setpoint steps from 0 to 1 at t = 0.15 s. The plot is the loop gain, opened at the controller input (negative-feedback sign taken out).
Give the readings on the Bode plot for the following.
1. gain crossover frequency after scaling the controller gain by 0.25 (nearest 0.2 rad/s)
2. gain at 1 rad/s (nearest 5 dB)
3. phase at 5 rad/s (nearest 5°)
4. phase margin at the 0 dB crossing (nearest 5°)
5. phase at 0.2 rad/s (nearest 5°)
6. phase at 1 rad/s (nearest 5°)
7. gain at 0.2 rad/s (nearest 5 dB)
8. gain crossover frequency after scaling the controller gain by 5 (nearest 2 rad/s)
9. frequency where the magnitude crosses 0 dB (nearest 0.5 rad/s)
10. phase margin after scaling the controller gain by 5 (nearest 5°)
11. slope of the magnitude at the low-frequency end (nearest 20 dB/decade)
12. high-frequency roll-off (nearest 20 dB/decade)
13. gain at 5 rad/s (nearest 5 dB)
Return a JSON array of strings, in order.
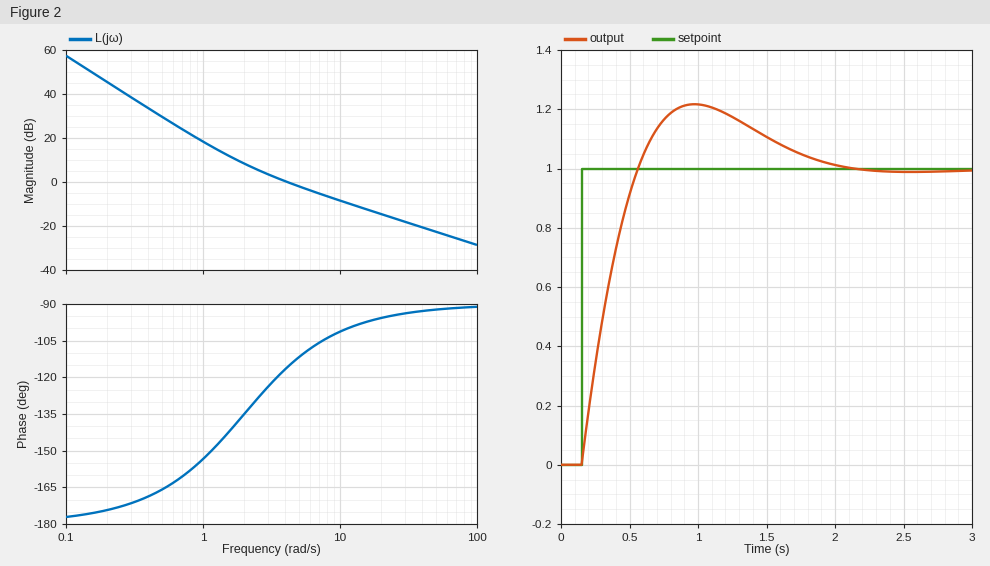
["1.6 rad/s", "20 dB", "-110°", "65°", "-175°", "-155°", "45 dB", "18 rad/s", "4.0 rad/s", "85°", "-40 dB/decade", "-20 dB/decade", "0 dB"]
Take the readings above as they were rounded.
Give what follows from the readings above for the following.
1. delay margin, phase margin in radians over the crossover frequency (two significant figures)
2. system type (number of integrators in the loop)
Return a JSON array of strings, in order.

["0.28 s", "2"]
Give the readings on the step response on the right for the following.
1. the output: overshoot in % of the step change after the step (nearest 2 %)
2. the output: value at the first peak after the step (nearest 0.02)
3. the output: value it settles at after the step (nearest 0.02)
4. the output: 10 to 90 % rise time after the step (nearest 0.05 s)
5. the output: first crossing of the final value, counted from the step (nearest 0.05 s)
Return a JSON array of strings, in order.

["22 %", "1.22", "1.00", "0.30 s", "0.40 s"]
